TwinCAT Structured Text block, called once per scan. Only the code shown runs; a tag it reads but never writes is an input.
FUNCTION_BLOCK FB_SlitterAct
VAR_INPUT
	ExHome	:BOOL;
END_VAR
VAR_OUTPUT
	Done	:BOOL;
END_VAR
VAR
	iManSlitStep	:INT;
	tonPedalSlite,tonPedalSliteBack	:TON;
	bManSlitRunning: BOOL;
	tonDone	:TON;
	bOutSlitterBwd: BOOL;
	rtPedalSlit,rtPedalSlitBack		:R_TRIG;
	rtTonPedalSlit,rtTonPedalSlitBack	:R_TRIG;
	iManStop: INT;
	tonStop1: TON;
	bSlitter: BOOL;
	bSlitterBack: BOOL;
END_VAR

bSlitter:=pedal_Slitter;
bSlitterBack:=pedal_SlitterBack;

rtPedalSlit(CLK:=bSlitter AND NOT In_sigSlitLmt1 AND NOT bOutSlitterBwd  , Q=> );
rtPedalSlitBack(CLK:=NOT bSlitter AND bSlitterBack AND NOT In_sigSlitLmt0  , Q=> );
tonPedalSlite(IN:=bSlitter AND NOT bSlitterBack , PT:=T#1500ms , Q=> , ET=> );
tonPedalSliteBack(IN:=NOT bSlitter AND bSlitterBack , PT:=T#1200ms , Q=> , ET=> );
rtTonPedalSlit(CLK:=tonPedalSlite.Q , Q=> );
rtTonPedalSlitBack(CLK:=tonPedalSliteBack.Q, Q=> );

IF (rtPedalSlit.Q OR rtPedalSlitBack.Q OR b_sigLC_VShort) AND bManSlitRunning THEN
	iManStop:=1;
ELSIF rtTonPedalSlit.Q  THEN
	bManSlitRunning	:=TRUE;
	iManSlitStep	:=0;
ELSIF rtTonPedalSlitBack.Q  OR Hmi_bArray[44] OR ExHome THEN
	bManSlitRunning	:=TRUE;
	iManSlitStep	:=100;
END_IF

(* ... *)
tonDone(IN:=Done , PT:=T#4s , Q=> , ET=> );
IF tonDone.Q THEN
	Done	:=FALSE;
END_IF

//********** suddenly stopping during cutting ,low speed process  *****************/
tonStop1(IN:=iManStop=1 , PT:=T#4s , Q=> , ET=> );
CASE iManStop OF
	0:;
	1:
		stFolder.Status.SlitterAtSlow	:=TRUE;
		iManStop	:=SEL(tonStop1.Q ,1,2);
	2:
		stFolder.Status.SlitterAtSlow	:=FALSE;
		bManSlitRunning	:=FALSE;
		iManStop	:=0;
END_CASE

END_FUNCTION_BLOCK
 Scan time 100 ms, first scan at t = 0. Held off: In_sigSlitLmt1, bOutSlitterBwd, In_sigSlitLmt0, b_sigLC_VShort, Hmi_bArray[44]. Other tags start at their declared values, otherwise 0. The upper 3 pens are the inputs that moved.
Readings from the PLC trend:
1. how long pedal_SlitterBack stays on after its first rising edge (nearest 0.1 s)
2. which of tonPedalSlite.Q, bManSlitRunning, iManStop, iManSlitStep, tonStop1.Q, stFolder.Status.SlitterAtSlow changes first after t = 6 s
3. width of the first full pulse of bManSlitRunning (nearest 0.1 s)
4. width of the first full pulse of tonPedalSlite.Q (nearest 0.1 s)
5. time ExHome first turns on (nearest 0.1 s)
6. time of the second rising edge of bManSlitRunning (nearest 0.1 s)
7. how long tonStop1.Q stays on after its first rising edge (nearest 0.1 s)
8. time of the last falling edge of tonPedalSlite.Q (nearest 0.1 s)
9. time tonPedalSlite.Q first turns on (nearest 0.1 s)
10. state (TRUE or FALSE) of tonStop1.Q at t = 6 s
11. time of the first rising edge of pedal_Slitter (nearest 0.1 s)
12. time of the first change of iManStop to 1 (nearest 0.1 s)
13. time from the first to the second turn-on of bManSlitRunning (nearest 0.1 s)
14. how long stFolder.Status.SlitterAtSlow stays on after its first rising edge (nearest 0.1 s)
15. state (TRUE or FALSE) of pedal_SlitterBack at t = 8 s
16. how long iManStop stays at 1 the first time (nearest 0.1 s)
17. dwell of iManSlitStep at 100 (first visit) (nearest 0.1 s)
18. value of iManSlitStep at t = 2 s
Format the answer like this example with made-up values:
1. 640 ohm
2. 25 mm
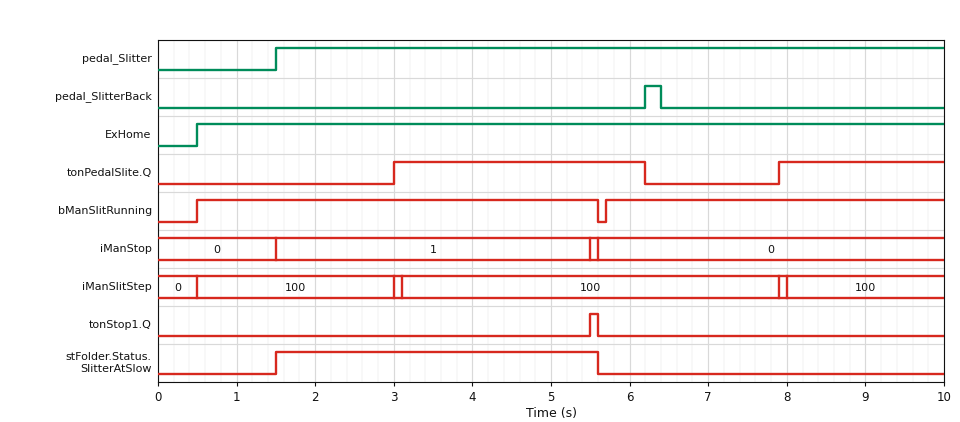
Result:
1. 0.2 s
2. tonPedalSlite.Q
3. 5.1 s
4. 3.2 s
5. 0.5 s
6. 5.7 s
7. 0.1 s
8. 6.2 s
9. 3.0 s
10. FALSE
11. 1.5 s
12. 1.5 s
13. 5.2 s
14. 4.1 s
15. FALSE
16. 4.0 s
17. 2.5 s
18. 100
